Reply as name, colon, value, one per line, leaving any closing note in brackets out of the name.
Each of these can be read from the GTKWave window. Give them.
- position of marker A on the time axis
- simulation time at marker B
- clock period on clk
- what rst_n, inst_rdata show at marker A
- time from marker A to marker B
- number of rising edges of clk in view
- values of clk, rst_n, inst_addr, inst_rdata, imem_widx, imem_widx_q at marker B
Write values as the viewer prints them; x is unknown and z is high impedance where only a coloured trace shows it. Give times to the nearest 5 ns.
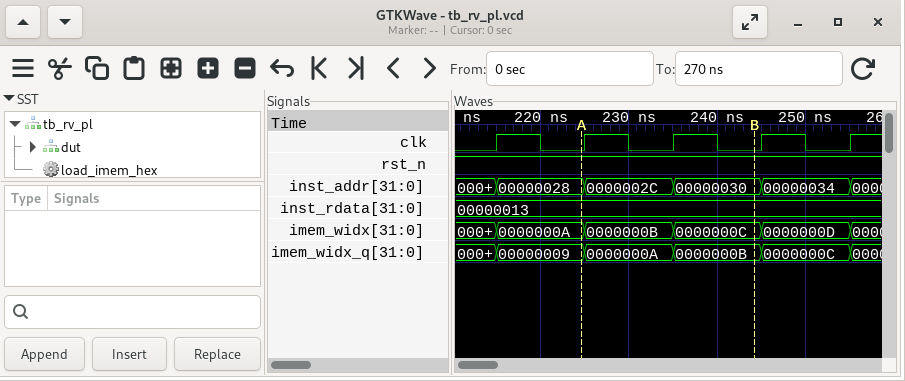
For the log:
position of marker A on the time axis: 225 ns
simulation time at marker B: 245 ns
clock period on clk: 10 ns
what rst_n, inst_rdata show at marker A: rst_n=1, inst_rdata=00000013
time from marker A to marker B: 20 ns
number of rising edges of clk in view: 5
values of clk, rst_n, inst_addr, inst_rdata, imem_widx, imem_widx_q at marker B: clk=0, rst_n=1, inst_addr=00000030, inst_rdata=00000013, imem_widx=0000000C, imem_widx_q=0000000B
